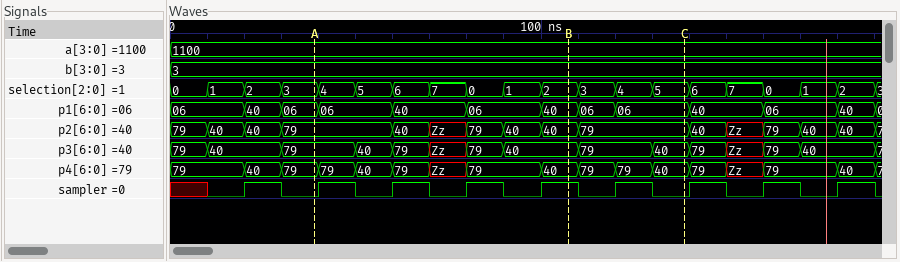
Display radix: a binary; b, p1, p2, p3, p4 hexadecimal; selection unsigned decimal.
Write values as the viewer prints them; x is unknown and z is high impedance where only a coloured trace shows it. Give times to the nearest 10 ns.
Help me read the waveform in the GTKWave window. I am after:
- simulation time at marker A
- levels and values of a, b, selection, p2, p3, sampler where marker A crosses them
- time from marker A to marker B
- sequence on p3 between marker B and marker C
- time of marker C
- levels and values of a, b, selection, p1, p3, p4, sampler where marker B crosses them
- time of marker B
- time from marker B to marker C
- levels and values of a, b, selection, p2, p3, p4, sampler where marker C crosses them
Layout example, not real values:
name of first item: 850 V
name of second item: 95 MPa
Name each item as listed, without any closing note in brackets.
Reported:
simulation time at marker A: 40 ns
levels and values of a, b, selection, p2, p3, sampler where marker A crosses them: a=1100, b=3, selection=3, p2=79, p3=79, sampler=0
time from marker A to marker B: 70 ns
sequence on p3 between marker B and marker C: 40, 79, 40
time of marker C: 140 ns
levels and values of a, b, selection, p1, p3, p4, sampler where marker B crosses them: a=1100, b=3, selection=2, p1=40, p3=40, p4=40, sampler=1
time of marker B: 110 ns
time from marker B to marker C: 30 ns
levels and values of a, b, selection, p2, p3, p4, sampler where marker C crosses them: a=1100, b=3, selection=5, p2=79, p3=40, p4=40, sampler=0
